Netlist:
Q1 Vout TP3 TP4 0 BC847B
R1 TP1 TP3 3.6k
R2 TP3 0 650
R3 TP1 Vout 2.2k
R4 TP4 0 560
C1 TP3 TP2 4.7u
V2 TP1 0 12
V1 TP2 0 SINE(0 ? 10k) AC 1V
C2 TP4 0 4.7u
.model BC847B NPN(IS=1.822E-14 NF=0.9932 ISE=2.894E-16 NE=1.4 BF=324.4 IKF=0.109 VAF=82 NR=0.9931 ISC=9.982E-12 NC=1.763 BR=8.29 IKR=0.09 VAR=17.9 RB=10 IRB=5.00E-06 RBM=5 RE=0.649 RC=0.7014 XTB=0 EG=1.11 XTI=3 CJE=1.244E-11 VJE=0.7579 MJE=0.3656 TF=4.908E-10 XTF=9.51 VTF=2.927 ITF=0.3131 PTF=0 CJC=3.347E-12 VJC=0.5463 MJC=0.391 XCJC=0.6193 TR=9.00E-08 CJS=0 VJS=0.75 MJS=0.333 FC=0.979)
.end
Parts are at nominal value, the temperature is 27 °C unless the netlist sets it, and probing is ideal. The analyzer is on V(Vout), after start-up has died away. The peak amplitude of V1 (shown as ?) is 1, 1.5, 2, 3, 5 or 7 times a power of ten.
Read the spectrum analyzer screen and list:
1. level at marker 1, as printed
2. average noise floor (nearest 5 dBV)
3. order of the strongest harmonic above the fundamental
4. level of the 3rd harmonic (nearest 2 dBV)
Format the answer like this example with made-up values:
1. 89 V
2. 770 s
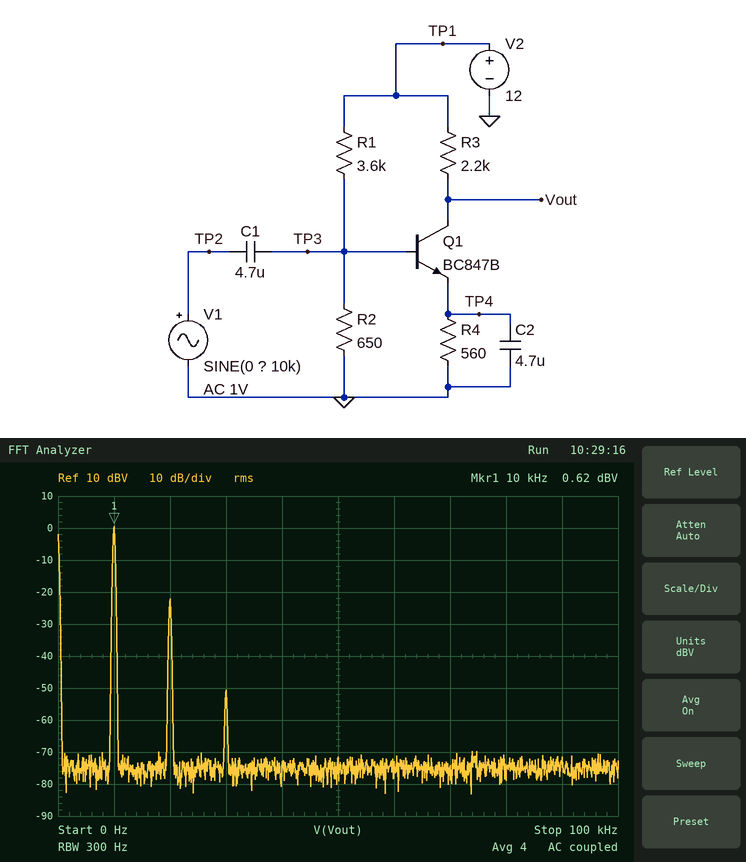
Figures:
1. 0.62 dBV
2. -75 dBV
3. 2
4. -50 dBV
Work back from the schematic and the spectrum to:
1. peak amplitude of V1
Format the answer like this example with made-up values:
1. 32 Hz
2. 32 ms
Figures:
1. 10 mV
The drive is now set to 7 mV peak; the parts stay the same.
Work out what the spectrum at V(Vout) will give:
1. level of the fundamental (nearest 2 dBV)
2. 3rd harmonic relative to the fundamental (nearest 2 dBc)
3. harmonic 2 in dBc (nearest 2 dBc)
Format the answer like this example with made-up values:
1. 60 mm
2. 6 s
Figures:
1. -2 dBV
2. -58 dBc
3. -26 dBc
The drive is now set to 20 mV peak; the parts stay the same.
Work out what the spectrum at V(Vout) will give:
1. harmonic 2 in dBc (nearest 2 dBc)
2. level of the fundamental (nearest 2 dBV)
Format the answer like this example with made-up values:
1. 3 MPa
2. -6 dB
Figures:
1. -16 dBc
2. 6 dBV
